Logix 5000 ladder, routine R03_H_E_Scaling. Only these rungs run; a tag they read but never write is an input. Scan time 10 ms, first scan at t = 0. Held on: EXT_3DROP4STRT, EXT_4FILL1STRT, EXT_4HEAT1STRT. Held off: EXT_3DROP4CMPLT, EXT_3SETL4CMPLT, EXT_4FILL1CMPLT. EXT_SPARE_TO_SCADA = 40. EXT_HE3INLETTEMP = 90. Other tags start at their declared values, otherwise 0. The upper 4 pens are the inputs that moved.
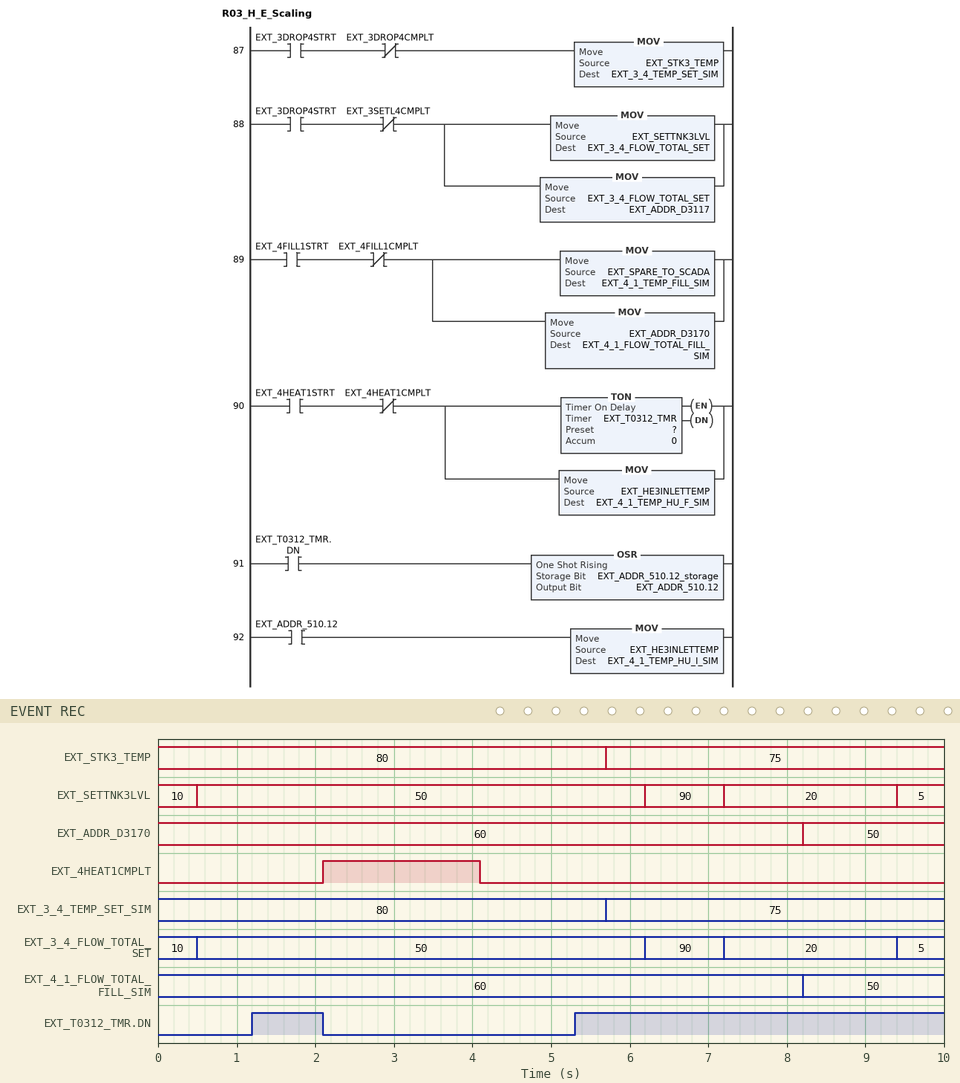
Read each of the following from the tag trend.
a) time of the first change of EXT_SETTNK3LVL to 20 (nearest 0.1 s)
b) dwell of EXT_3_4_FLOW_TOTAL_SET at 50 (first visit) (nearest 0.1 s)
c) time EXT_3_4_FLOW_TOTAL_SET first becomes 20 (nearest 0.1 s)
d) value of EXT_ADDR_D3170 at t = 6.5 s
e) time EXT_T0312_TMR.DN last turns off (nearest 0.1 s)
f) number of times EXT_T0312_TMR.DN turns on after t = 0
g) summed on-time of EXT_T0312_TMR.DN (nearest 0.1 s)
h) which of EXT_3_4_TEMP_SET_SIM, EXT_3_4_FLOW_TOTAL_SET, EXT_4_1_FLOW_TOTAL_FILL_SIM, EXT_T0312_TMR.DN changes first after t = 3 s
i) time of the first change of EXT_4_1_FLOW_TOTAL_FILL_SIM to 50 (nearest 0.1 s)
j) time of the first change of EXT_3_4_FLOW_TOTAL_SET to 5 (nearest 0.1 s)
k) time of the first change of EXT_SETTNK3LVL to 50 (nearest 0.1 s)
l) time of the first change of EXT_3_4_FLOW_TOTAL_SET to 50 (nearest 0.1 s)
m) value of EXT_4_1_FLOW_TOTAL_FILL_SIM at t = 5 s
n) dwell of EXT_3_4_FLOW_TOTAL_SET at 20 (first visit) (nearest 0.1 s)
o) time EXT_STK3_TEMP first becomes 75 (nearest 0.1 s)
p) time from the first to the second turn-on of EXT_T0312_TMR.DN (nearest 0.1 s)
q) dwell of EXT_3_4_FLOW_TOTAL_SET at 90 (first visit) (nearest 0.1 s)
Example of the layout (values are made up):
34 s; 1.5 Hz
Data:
7.2 s; 5.7 s; 7.2 s; 60; 2.1 s; 2; 5.6 s; EXT_T0312_TMR.DN; 8.2 s; 9.4 s; 0.5 s; 0.5 s; 60; 2.2 s; 5.7 s; 4.1 s; 1.0 s
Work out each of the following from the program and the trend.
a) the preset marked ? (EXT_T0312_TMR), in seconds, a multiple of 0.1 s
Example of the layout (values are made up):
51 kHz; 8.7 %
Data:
1.2 s
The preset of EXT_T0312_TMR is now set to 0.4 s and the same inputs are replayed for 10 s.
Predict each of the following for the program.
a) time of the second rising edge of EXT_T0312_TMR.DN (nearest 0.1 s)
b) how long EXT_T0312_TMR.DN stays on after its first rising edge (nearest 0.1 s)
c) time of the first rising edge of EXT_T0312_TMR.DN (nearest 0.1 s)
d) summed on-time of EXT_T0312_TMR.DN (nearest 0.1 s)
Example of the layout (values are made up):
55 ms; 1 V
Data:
4.5 s; 1.7 s; 0.4 s; 7.2 s
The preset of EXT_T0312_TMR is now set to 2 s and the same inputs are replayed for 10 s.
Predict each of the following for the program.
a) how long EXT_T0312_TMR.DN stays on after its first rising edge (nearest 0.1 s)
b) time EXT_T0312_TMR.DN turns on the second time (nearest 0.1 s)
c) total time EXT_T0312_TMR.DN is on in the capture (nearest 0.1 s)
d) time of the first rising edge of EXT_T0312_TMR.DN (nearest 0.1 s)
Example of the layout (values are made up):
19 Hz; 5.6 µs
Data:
0.1 s; 6.1 s; 4.0 s; 2.0 s
